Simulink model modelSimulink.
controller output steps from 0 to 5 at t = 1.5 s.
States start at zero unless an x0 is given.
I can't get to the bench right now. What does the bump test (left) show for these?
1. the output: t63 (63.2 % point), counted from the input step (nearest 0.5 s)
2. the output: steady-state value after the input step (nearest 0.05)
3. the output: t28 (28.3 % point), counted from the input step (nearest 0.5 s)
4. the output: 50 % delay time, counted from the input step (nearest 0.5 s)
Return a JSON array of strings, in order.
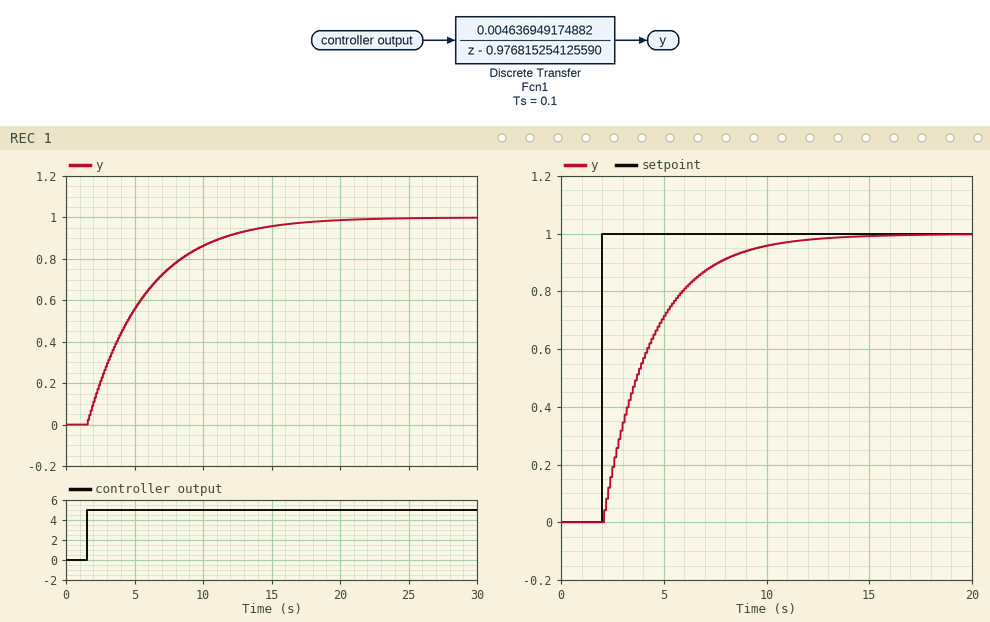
["4.5 s", "1.00", "1.5 s", "3.0 s"]
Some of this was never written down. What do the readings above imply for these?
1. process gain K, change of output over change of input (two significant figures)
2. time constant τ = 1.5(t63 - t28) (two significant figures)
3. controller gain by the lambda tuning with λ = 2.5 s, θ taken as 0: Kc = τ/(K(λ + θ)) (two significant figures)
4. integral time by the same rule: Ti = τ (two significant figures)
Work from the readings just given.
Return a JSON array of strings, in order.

["0.20", "4.5 s", "9.0", "4.5 s"]
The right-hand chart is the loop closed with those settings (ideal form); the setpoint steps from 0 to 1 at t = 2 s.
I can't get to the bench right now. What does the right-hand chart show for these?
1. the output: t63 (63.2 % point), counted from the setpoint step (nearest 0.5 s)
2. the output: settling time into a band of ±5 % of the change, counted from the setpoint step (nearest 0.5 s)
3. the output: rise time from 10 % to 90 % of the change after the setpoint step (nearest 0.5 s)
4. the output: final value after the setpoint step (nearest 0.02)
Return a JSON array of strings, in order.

["2.5 s", "7.5 s", "5.5 s", "1.00"]
